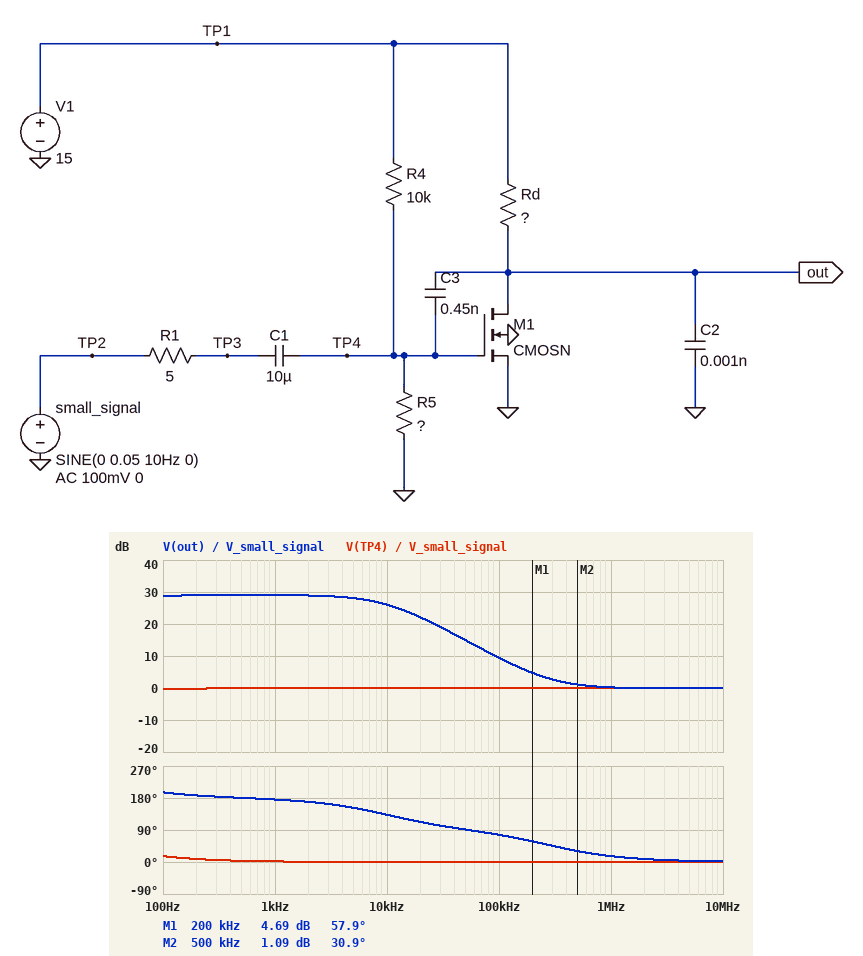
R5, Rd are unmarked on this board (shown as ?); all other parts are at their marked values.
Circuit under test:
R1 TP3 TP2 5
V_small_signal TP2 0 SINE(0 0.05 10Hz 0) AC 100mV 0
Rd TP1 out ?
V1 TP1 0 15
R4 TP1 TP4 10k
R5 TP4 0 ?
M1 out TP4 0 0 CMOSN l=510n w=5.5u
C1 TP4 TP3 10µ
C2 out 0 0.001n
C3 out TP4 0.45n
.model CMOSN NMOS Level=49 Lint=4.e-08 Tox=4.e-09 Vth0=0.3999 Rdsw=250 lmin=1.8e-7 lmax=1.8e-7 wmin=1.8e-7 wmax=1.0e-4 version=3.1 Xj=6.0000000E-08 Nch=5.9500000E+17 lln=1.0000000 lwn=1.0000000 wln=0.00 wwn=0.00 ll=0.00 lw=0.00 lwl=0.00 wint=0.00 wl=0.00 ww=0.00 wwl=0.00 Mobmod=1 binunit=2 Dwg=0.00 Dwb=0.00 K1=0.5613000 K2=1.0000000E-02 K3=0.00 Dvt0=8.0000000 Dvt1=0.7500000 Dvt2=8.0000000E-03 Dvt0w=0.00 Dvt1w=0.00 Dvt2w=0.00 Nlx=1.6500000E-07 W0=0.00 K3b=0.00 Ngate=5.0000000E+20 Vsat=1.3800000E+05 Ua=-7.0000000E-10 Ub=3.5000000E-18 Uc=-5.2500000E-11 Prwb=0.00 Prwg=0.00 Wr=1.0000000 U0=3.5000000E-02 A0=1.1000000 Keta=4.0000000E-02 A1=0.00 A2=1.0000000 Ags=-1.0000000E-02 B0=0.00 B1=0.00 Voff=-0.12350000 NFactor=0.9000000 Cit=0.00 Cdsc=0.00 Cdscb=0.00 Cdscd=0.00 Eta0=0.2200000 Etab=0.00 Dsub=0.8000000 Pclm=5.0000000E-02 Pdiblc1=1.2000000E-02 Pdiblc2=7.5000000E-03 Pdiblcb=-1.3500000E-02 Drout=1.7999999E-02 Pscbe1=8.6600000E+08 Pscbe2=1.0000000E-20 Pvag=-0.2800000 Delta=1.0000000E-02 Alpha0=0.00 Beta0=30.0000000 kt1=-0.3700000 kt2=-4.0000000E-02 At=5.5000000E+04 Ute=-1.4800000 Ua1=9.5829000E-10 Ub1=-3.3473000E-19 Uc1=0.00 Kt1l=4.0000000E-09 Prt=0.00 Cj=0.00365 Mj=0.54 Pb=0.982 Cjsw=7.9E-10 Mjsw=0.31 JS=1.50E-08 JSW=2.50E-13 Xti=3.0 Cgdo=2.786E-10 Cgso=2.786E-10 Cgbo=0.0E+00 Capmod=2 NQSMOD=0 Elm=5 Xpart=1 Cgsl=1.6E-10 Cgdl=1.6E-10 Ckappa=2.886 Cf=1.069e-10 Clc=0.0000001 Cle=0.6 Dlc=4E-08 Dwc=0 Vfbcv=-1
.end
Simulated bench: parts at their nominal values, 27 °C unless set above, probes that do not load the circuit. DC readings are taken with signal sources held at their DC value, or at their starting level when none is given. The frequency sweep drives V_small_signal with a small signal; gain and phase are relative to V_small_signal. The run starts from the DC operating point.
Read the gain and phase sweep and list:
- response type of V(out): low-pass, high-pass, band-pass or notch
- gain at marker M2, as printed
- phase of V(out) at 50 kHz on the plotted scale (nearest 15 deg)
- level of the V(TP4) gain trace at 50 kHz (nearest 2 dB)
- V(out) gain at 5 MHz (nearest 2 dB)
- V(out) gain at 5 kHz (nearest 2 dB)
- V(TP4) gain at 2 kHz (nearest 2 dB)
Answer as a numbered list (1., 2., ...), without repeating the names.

1. low-pass
2. 1.09 dB
3. 90 deg
4. 0 dB
5. 0 dB
6. 28 dB
7. 0 dB
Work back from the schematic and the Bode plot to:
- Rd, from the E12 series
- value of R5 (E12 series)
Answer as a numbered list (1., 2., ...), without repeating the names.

1. 82 kΩ
2. 560 Ω
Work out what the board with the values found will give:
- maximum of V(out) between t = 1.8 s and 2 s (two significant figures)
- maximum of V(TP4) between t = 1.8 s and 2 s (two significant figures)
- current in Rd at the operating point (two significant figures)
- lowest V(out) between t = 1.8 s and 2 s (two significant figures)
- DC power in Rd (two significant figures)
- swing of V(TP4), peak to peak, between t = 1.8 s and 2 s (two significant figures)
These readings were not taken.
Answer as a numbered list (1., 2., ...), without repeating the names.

1. 2.5 V
2. 810 mV
3. 160 µA
4. 1.6 V
5. 2.0 mW
6. 32 mV
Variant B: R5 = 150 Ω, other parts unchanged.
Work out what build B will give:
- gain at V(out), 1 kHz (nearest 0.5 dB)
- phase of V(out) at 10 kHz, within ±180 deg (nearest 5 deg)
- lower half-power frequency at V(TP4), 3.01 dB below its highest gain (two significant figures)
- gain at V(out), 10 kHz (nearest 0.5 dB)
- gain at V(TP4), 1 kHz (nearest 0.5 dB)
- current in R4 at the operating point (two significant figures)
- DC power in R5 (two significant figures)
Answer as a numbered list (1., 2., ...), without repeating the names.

1. -13.0 dB
2. 25 deg
3. 100 Hz
4. -1.0 dB
5. -0.5 dB
6. 1.5 mA
7. 330 µW
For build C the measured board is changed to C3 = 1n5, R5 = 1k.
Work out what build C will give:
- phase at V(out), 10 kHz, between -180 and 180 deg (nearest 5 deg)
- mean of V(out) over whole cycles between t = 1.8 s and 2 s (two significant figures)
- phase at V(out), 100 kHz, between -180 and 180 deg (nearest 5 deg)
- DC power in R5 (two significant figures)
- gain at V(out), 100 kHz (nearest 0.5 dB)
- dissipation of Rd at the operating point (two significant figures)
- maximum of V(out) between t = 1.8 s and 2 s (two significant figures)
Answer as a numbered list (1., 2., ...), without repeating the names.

1. 140 deg
2. 95 mV
3. 70 deg
4. 1.9 mW
5. -6.5 dB
6. 2.7 mW
7. 97 mV
